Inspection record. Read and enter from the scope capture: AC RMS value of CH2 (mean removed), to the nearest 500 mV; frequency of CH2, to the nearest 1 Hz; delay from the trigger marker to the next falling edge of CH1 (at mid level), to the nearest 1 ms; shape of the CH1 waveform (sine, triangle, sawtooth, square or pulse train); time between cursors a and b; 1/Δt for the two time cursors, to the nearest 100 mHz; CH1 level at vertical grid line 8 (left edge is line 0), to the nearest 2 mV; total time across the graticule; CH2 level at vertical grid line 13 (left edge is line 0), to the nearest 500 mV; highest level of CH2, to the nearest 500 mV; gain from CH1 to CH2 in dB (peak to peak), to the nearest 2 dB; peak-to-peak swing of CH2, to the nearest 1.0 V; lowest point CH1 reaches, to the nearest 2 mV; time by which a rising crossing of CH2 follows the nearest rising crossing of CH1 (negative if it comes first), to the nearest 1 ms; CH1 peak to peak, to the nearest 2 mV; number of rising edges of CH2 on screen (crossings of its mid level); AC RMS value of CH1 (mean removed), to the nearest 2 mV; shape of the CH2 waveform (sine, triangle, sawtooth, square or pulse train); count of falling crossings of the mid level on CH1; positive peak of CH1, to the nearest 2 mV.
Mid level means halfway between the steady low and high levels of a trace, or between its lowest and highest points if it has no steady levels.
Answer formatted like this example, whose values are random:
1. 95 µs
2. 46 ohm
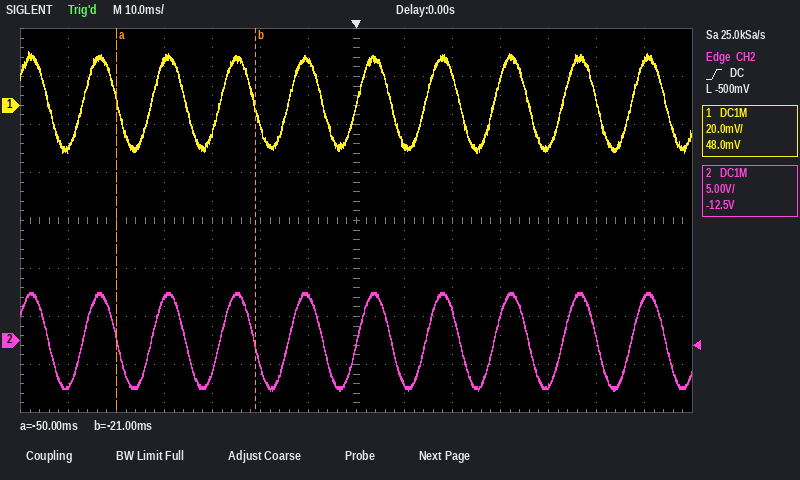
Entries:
1. 3.5 V
2. 70 Hz
3. 7 ms
4. sine
5. 29 ms
6. 34.5 Hz
7. -16 mV
8. 140 ms
9. 4.5 V
10. 5.0 V
11. 48 dB
12. 10.0 V
13. -20 mV
14. 0 ms
15. 42 mV
16. 9
17. 14 mV
18. sine
19. 10
20. 22 mV
